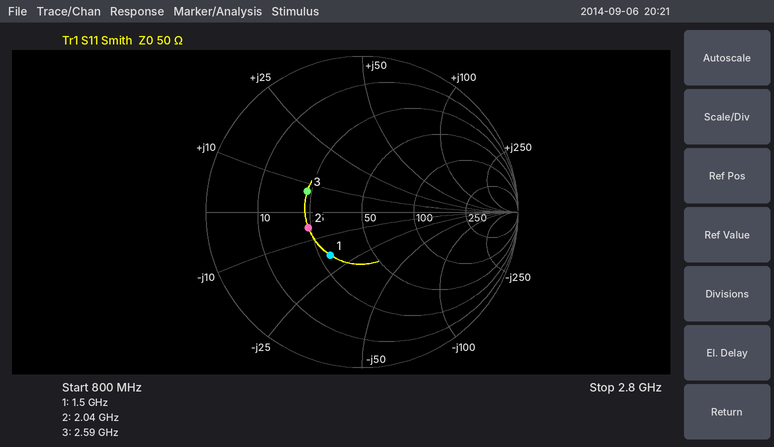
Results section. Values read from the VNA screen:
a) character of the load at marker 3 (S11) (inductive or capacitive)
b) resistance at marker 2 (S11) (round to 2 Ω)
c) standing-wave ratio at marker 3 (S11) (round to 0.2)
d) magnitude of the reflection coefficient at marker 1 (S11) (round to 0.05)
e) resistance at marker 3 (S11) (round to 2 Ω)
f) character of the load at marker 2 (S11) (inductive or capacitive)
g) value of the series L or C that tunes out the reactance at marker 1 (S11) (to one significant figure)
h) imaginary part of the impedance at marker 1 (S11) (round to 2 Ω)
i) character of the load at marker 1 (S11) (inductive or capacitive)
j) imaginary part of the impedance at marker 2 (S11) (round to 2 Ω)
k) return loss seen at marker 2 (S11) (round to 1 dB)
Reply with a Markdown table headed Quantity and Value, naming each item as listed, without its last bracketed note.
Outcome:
| Quantity | Value |
|---|---|
| character of the load at marker 3 (S11) | inductive |
| resistance at marker 2 (S11) | 24 Ω |
| standing-wave ratio at marker 3 (S11) | 2.2 |
| magnitude of the reflection coefficient at marker 1 (S11) | 0.35 |
| resistance at marker 3 (S11) | 24 Ω |
| character of the load at marker 2 (S11) | capacitive |
| value of the series L or C that tunes out the reactance at marker 1 (S11) | 2 nH |
| imaginary part of the impedance at marker 1 (S11) | -18 Ω |
| character of the load at marker 1 (S11) | capacitive |
| imaginary part of the impedance at marker 2 (S11) | -6 Ω |
| return loss seen at marker 2 (S11) | 9 dB |
